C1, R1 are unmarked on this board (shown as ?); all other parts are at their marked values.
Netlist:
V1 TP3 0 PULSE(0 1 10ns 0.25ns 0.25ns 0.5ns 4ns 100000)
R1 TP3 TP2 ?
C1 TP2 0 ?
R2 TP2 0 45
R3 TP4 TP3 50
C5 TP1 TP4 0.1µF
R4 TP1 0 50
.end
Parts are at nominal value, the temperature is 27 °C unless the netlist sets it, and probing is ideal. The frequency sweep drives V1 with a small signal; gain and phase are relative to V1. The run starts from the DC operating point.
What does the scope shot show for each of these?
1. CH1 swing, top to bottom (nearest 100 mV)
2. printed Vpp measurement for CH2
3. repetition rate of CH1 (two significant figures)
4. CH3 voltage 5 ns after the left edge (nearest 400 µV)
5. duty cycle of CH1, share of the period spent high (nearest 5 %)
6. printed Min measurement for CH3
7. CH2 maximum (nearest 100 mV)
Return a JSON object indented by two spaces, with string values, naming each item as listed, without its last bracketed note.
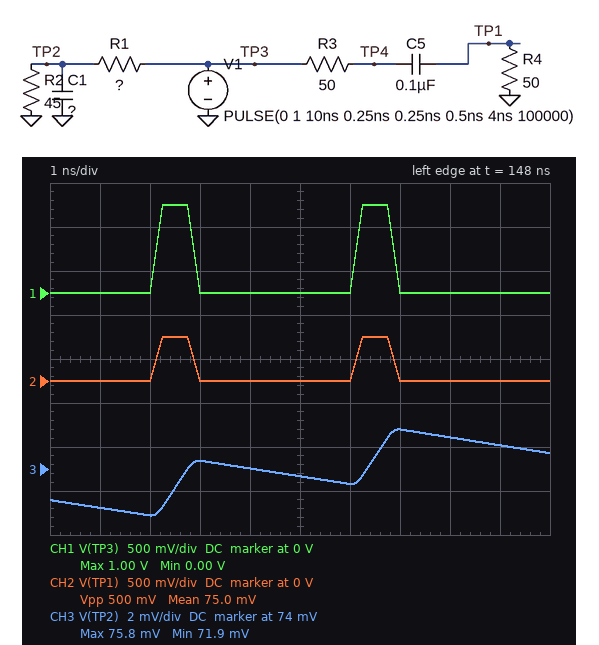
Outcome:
{
  "CH1 swing, top to bottom": "1.0 V",
  "printed Vpp measurement for CH2": "500 mV",
  "repetition rate of CH1": "250 MHz",
  "CH3 voltage 5 ns after the left edge": "73.6 mV",
  "duty cycle of CH1, share of the period spent high": "20 %",
  "printed Min measurement for CH3": "71.9 mV",
  "CH2 maximum": "500 mV"
}
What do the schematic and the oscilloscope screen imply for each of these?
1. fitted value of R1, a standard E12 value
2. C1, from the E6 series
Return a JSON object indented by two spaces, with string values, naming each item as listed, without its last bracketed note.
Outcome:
{
  "fitted value of R1, a standard E12 value": "12 Ω",
  "C1, from the E6 series": "22 nF"
}
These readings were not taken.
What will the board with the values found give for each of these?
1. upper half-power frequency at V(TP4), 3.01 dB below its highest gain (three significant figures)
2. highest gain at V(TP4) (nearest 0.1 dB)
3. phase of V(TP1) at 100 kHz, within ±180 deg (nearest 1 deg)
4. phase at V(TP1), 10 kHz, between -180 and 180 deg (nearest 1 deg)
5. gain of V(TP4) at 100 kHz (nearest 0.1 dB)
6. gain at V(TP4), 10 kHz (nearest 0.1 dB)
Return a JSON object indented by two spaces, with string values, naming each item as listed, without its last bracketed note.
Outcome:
{
  "upper half-power frequency at V(TP4), 3.01 dB below its highest gain": "22.5 kHz",
  "highest gain at V(TP4)": "0 dB",
  "phase of V(TP1) at 100 kHz, within ±180 deg": "9 deg",
  "phase at V(TP1), 10 kHz, between -180 and 180 deg": "58 deg",
  "gain of V(TP4) at 100 kHz": "-5.7 dB",
  "gain at V(TP4), 10 kHz": "-1.0 dB"
}
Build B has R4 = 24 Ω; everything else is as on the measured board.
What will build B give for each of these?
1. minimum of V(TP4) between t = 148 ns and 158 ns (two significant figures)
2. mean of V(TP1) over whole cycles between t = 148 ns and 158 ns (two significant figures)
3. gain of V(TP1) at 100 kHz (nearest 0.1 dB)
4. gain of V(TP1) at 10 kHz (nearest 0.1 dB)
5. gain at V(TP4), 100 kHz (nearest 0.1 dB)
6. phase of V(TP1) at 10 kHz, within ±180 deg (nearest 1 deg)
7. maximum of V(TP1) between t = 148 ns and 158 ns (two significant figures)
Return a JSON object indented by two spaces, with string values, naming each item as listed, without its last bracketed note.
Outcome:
{
  "minimum of V(TP4) between t = 148 ns and 158 ns": "2.4 mV",
  "mean of V(TP1) over whole cycles between t = 148 ns and 158 ns": "60 mV",
  "gain of V(TP1) at 100 kHz": "-10.0 dB",
  "gain of V(TP1) at 10 kHz": "-17.3 dB",
  "gain at V(TP4), 100 kHz": "-8.4 dB",
  "phase of V(TP1) at 10 kHz, within ±180 deg": "65 deg",
  "maximum of V(TP1) between t = 148 ns and 158 ns": "320 mV"
}
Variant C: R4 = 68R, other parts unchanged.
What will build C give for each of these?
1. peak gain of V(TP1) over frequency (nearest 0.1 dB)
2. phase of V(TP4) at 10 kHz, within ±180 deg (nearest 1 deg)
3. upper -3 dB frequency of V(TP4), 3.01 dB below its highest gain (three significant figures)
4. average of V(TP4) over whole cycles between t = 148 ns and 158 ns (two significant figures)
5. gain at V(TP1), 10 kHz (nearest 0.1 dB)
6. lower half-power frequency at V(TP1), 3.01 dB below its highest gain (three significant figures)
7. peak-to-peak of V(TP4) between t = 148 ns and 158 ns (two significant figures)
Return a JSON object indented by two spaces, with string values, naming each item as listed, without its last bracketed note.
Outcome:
{
  "peak gain of V(TP1) over frequency": "-4.8 dB",
  "phase of V(TP4) at 10 kHz, within ±180 deg": "-13 deg",
  "upper -3 dB frequency of V(TP4), 3.01 dB below its highest gain": "23.3 kHz",
  "average of V(TP4) over whole cycles between t = 148 ns and 158 ns": "110 mV",
  "gain at V(TP1), 10 kHz": "-9.3 dB",
  "lower half-power frequency at V(TP1), 3.01 dB below its highest gain": "13.5 kHz",
  "peak-to-peak of V(TP4) between t = 148 ns and 158 ns": "580 mV"
}
